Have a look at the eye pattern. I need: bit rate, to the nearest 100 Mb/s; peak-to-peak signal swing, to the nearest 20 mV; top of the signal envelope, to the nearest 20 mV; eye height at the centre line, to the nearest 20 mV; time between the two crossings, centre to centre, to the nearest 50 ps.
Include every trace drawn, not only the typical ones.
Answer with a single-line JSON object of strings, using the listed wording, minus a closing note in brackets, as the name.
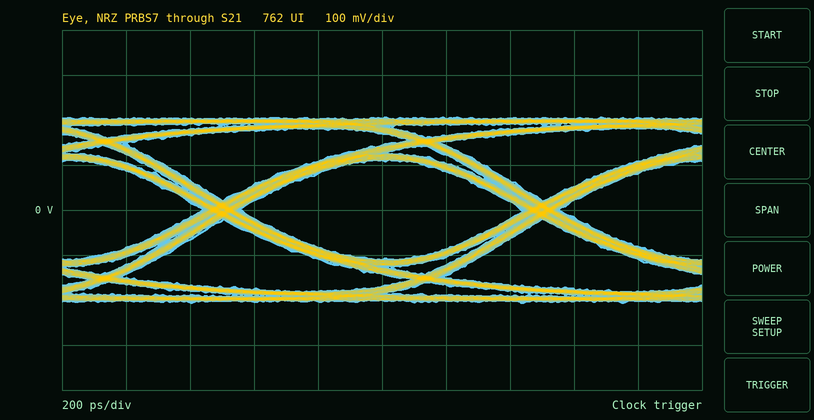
{"bit rate, to the nearest 100 Mb/s": "1.0 Gb/s", "peak-to-peak signal swing, to the nearest 20 mV": "420 mV", "top of the signal envelope, to the nearest 20 mV": "200 mV", "eye height at the centre line, to the nearest 20 mV": "220 mV", "time between the two crossings, centre to centre, to the nearest 50 ps": "1.00 ns"}
